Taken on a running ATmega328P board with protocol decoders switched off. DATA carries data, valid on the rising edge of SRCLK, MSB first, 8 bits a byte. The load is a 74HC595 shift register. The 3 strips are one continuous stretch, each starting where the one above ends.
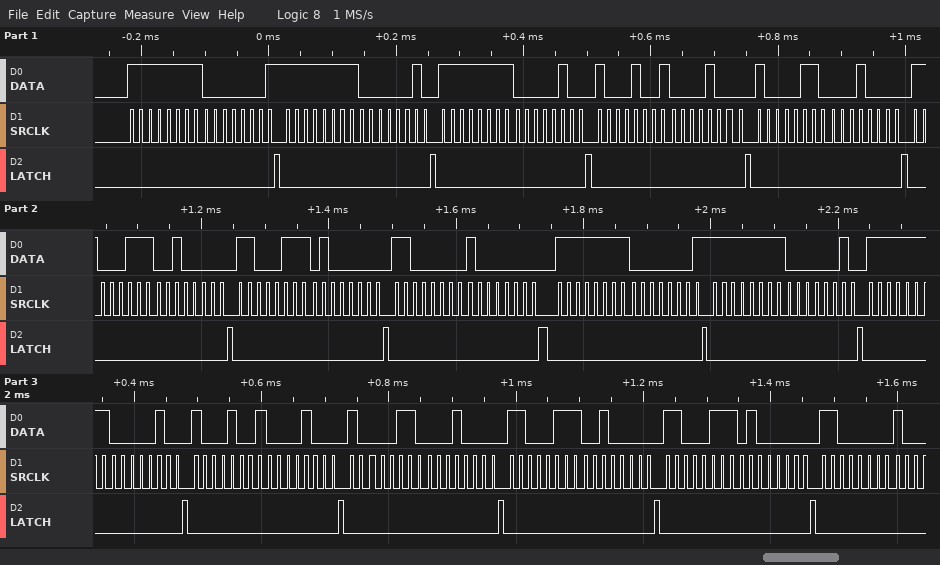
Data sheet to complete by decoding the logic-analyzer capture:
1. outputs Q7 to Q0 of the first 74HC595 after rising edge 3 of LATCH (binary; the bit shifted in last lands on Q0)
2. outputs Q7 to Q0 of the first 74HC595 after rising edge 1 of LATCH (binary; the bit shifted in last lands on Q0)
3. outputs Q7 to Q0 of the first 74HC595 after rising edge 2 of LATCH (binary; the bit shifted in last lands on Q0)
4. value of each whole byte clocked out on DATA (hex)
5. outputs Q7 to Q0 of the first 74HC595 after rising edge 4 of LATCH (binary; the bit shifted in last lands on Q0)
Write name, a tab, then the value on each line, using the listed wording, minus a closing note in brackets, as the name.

outputs Q7 to Q0 of the first 74HC595 after rising edge 3 of LATCH	00000100
outputs Q7 to Q0 of the first 74HC595 after rising edge 1 of LATCH	00000001
outputs Q7 to Q0 of the first 74HC595 after rising edge 2 of LATCH	00000010
value of each whole byte clocked out on DATA	0xFF 0x01 0xFF 0x02 0xFF 0x04 0x89 0x08 0x86 0x10 0xC7 0x20 0xC7 0x40 0xC0 0x80 0xFF 0x01 0xFF 0x02 0xFF 0x04 0x89 0x08 0x86 0x10 0xC7 0x20 0xC7 0x40 0xC0
outputs Q7 to Q0 of the first 74HC595 after rising edge 4 of LATCH	00001000
